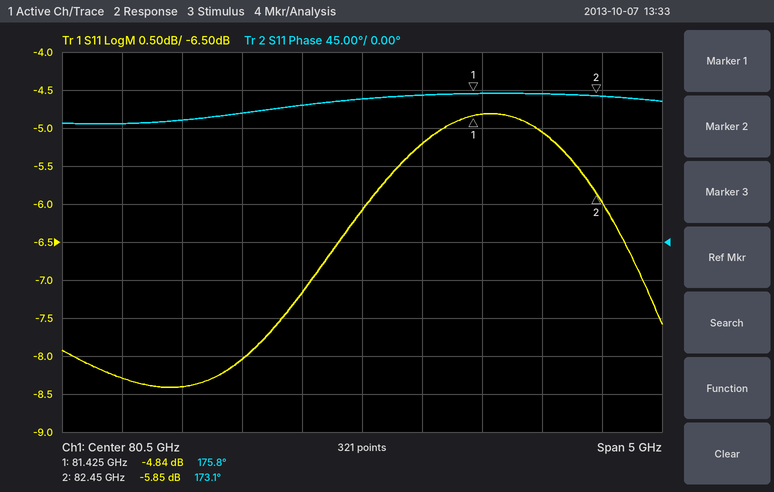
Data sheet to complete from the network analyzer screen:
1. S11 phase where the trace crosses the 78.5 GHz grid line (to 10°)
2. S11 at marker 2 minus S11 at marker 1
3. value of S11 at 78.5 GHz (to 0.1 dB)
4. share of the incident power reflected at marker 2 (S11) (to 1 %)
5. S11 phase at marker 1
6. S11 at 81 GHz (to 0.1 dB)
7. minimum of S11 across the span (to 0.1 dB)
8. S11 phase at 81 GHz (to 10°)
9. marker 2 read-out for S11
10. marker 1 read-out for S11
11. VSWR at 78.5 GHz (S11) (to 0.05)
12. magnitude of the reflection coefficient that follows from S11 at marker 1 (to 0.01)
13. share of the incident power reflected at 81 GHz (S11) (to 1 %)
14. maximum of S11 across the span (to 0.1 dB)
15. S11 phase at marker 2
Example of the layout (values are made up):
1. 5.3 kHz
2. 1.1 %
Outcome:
1. 140°
2. -1.01 dB
3. -8.3 dB
4. 26 %
5. 175.8°
6. -5.2 dB
7. -8.4 dB
8. 170°
9. -5.85 dB
10. -4.84 dB
11. 2.25
12. 0.57
13. 30 %
14. -4.8 dB
15. 173.1°
